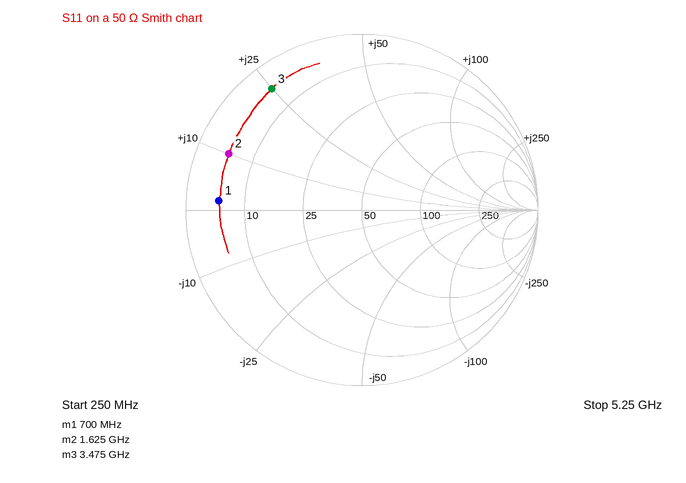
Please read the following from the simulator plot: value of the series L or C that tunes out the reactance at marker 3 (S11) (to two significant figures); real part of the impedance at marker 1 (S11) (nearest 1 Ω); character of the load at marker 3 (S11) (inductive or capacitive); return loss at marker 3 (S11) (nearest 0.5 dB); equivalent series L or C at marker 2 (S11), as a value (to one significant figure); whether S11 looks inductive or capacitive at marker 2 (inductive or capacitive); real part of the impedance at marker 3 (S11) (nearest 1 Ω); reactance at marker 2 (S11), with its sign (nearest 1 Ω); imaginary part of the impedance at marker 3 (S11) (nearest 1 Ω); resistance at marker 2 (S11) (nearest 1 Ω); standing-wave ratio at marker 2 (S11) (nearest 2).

1.8 pF
5 Ω
inductive
1.5 dB
1.0 nH
inductive
5 Ω
+10 Ω
+25 Ω
5 Ω
10
